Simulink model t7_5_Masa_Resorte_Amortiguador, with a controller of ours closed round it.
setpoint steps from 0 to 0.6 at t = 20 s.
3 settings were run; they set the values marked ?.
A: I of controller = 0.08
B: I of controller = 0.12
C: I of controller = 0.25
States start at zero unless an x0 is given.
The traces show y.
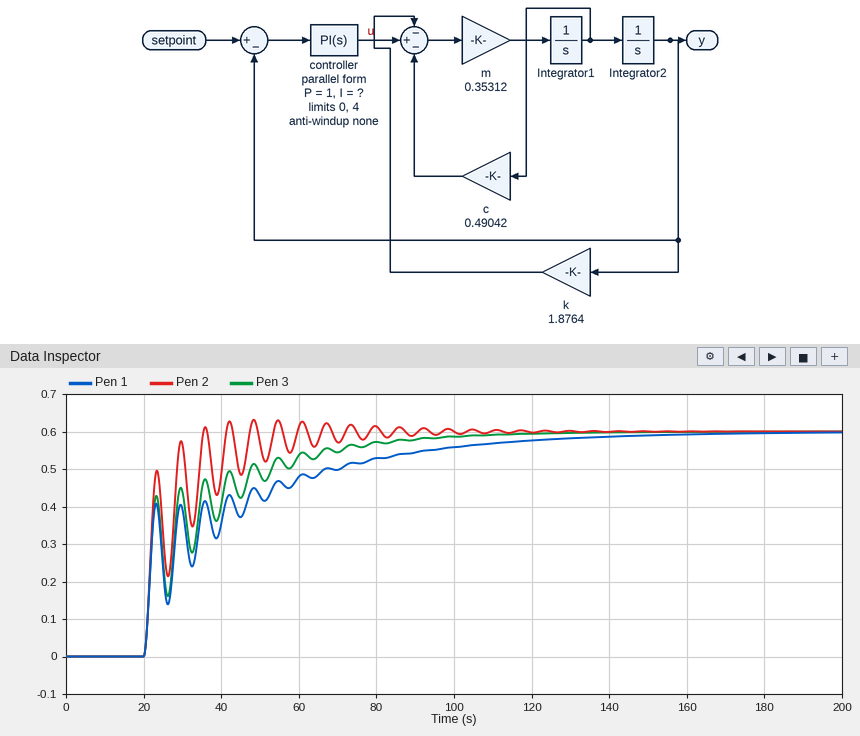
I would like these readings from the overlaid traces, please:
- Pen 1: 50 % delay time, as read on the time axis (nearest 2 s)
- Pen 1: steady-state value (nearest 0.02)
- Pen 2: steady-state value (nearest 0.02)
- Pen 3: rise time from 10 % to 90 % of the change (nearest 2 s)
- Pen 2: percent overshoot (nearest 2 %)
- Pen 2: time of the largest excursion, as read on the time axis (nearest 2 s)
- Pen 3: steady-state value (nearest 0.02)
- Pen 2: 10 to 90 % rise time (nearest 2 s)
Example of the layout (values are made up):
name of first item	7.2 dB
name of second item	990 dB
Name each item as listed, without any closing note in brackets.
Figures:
Pen 1: 50 % delay time, as read on the time axis	22 s
Pen 1: steady-state value	0.60
Pen 2: steady-state value	0.60
Pen 3: rise time from 10 % to 90 % of the change	40 s
Pen 2: percent overshoot	6 %
Pen 2: time of the largest excursion, as read on the time axis	48 s
Pen 3: steady-state value	0.60
Pen 2: 10 to 90 % rise time	8 s
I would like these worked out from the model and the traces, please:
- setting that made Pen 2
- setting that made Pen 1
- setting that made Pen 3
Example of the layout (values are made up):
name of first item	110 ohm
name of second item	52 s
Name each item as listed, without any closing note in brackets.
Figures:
setting that made Pen 2	C
setting that made Pen 1	A
setting that made Pen 3	B
